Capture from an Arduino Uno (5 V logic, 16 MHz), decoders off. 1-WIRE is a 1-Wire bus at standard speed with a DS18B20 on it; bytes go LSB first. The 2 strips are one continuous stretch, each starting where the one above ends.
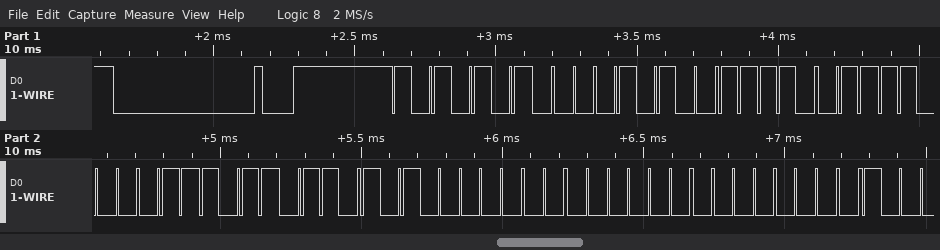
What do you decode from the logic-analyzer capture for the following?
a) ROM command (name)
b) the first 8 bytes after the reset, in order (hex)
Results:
Match ROM
55 28 CF C3 6D 05 00 00
